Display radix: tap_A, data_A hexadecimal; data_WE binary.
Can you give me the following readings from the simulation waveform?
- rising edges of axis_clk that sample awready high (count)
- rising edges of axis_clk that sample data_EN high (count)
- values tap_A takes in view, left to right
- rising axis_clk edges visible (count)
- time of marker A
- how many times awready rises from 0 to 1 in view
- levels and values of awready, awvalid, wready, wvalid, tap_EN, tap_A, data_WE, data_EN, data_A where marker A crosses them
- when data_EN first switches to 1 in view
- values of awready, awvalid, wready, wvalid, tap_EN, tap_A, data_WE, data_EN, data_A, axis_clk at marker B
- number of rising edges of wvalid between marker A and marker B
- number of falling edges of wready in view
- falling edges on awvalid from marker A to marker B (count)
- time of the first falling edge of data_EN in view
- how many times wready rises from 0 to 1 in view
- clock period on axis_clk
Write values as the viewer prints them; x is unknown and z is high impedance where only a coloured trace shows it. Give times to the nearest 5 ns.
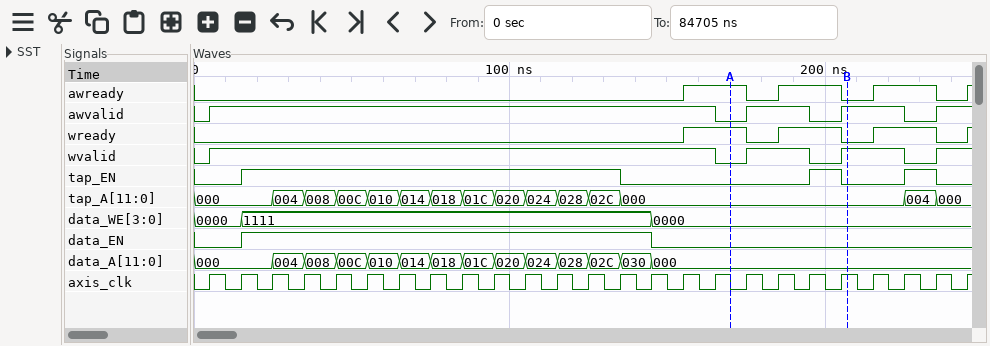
6
13
000, 004, 008, 00C, 010, 014, 018, 01C, 020, 024, 028, 02C, 000, 004, 000
25
170 ns
4
awready=1, awvalid=0, wready=1, wvalid=0, tap_EN=0, tap_A=000, data_WE=0000, data_EN=0, data_A=000
15 ns
awready=0, awvalid=1, wready=0, wvalid=1, tap_EN=0, tap_A=000, data_WE=0000, data_EN=0, data_A=000, axis_clk=1
2
3
1
145 ns
4
10 ns
